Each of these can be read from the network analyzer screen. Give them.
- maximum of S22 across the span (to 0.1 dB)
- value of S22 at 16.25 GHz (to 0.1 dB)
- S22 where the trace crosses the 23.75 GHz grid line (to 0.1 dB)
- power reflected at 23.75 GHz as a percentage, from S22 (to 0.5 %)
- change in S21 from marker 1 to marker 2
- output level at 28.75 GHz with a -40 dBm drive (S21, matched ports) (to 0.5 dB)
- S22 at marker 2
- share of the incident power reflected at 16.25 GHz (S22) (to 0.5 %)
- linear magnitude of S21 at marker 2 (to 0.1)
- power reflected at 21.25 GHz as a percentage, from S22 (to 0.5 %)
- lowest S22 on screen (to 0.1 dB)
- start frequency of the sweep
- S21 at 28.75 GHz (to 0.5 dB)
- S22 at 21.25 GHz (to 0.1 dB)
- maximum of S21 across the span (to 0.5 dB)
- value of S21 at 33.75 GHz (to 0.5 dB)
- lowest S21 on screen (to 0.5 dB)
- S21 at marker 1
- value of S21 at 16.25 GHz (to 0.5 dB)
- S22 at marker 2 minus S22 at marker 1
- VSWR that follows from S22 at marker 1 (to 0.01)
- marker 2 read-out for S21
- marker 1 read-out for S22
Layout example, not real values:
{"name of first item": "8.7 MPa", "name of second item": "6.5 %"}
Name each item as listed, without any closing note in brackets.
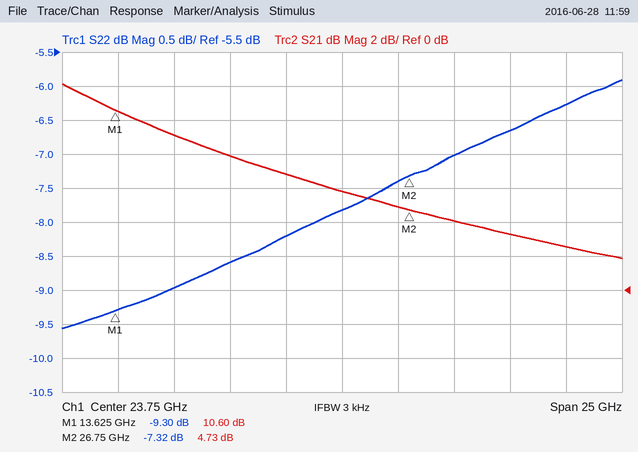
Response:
{"maximum of S22 across the span": "-5.9 dB", "value of S22 at 16.25 GHz": "-9.0 dB", "S22 where the trace crosses the 23.75 GHz grid line": "-7.8 dB", "power reflected at 23.75 GHz as a percentage, from S22": "16.5 %", "change in S21 from marker 1 to marker 2": "-5.87 dB", "output level at 28.75 GHz with a -40 dBm drive (S21, matched ports)": "-36.0 dBm", "S22 at marker 2": "-7.32 dB", "share of the incident power reflected at 16.25 GHz (S22)": "12.5 %", "linear magnitude of S21 at marker 2": "1.7", "power reflected at 21.25 GHz as a percentage, from S22": "15.0 %", "lowest S22 on screen": "-9.6 dB", "start frequency of the sweep": "11.25 GHz", "S21 at 28.75 GHz": "4.0 dB", "S22 at 21.25 GHz": "-8.2 dB", "maximum of S21 across the span": "12.0 dB", "value of S21 at 33.75 GHz": "2.5 dB", "lowest S21 on screen": "2.0 dB", "S21 at marker 1": "10.60 dB", "value of S21 at 16.25 GHz": "9.0 dB", "S22 at marker 2 minus S22 at marker 1": "1.98 dB", "VSWR that follows from S22 at marker 1": "2.04", "marker 2 read-out for S21": "4.73 dB", "marker 1 read-out for S22": "-9.30 dB"}
